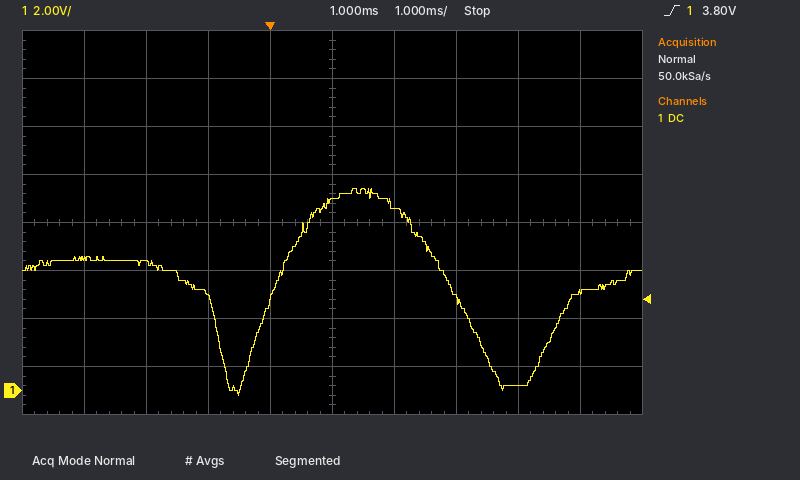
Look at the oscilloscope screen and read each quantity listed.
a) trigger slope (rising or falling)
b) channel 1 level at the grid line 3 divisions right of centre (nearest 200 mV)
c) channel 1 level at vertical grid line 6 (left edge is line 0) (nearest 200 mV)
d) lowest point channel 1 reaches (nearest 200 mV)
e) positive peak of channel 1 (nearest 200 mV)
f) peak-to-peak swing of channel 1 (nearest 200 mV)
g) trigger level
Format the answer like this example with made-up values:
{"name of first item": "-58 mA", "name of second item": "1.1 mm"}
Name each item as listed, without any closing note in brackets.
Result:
{"trigger slope": "rising", "channel 1 level at the grid line 3 divisions right of centre": "200 mV", "channel 1 level at vertical grid line 6 (left edge is line 0)": "7.6 V", "lowest point channel 1 reaches": "-200 mV", "positive peak of channel 1": "8.4 V", "peak-to-peak swing of channel 1": "8.6 V", "trigger level": "3.80 V"}
